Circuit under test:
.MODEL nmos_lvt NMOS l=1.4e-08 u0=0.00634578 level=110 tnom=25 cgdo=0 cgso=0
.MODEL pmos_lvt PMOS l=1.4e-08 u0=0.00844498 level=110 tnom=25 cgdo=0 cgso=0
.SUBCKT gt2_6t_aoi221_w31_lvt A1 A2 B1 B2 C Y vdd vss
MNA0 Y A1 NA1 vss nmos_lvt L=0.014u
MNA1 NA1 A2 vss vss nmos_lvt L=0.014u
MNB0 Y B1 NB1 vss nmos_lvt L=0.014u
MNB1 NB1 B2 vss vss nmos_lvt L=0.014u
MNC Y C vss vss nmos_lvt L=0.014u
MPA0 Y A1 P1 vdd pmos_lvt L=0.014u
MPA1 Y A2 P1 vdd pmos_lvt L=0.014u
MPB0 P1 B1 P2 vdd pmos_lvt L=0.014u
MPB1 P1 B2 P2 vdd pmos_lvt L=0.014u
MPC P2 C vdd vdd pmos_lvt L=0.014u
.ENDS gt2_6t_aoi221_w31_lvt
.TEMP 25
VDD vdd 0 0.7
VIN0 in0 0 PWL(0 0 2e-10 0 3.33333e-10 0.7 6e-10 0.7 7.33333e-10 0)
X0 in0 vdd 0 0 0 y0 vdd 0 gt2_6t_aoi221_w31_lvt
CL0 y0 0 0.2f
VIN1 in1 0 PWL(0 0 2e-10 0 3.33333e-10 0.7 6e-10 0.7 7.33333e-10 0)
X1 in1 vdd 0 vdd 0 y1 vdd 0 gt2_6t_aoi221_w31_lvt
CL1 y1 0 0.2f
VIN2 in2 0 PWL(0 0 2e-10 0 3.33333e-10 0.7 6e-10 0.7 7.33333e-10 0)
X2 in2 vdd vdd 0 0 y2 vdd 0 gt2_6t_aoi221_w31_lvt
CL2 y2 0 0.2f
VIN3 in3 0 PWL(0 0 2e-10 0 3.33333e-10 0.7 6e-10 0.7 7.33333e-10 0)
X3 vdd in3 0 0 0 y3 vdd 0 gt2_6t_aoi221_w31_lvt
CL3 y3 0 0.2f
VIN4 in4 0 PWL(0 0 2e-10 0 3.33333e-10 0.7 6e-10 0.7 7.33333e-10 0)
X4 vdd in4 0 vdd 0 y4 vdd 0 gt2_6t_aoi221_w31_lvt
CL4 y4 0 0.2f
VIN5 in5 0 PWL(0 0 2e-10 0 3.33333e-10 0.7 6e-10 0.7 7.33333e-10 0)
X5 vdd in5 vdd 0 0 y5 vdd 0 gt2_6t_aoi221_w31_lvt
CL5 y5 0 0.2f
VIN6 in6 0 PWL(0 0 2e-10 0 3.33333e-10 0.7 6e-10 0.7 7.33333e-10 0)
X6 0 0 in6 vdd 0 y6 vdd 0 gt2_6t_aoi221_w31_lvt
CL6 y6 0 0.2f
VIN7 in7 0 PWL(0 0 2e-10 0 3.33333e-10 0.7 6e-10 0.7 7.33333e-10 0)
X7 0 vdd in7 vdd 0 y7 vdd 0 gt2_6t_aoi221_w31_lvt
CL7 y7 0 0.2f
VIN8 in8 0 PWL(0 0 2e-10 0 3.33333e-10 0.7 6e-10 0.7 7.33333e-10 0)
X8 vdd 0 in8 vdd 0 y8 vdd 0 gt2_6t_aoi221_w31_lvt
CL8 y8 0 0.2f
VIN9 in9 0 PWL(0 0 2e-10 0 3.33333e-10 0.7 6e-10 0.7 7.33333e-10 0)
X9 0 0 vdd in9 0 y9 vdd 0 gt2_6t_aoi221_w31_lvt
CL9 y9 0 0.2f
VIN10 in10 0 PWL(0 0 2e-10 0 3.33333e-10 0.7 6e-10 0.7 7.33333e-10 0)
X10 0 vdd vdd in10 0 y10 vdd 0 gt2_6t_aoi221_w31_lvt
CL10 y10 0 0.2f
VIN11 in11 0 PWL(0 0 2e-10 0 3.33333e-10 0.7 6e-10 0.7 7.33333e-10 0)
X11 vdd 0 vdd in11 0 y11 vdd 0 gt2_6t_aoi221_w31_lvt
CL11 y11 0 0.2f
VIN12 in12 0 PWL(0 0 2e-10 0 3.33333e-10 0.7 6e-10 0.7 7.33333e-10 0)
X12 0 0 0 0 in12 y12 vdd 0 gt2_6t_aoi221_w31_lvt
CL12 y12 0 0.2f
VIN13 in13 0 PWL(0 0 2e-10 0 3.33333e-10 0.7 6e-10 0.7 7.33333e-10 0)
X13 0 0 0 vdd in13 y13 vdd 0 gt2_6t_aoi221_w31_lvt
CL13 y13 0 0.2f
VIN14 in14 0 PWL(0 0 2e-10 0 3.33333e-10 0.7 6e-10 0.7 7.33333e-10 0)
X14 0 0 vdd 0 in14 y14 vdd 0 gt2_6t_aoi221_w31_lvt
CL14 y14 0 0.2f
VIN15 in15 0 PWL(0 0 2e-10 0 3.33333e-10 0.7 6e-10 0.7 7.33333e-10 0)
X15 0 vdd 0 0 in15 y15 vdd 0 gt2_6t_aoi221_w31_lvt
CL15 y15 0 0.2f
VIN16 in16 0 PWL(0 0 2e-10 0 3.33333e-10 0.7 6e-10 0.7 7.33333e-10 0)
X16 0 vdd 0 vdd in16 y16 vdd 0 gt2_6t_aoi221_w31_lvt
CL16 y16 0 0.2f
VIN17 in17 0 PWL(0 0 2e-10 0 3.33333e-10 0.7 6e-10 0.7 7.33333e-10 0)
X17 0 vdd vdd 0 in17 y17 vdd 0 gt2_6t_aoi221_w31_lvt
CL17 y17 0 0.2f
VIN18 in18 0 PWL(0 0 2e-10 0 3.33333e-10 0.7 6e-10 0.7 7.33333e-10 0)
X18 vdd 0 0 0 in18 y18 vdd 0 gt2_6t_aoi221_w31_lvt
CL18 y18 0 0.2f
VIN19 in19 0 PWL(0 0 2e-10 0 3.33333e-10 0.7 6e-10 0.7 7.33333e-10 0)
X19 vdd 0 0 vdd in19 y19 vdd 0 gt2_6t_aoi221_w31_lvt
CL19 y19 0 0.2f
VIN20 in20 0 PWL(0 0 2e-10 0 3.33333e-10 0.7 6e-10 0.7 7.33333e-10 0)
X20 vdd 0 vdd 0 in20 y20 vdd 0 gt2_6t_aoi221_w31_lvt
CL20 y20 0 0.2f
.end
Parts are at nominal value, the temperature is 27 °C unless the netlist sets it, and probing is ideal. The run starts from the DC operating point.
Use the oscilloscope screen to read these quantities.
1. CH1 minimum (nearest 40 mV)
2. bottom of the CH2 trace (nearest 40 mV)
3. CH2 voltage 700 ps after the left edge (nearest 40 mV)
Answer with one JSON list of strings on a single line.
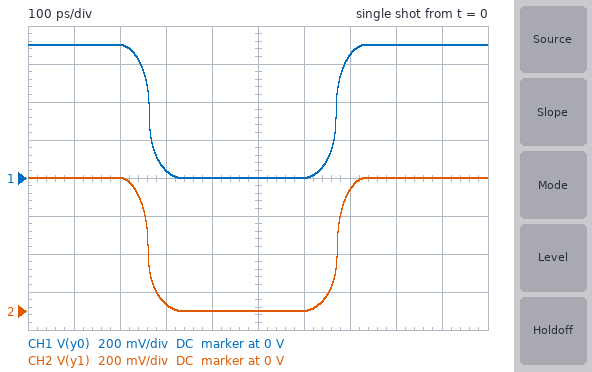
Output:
["0 V", "0 V", "640 mV"]
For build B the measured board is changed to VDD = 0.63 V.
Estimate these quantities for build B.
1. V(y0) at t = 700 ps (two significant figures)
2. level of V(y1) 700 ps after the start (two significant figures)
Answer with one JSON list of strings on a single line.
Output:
["570 mV", "560 mV"]
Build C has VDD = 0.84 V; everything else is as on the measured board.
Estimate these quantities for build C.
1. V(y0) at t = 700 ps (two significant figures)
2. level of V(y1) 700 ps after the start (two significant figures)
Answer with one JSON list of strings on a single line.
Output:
["800 mV", "790 mV"]
